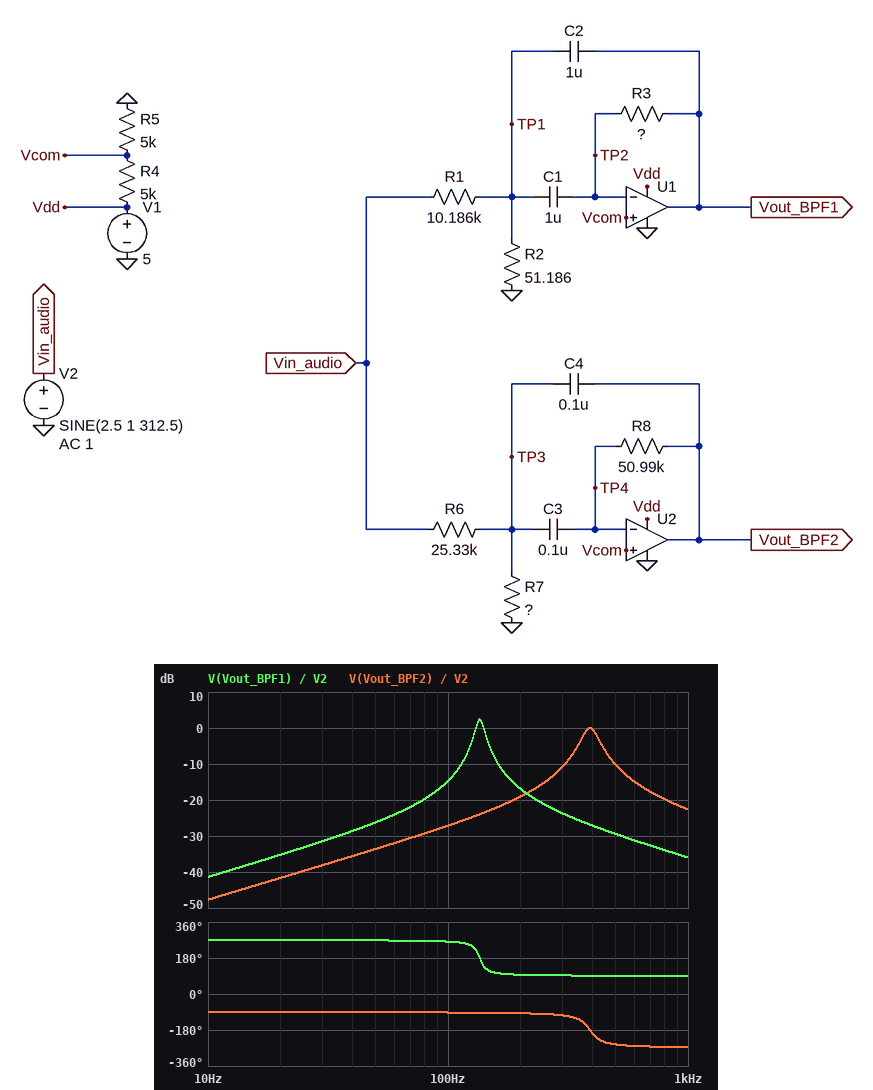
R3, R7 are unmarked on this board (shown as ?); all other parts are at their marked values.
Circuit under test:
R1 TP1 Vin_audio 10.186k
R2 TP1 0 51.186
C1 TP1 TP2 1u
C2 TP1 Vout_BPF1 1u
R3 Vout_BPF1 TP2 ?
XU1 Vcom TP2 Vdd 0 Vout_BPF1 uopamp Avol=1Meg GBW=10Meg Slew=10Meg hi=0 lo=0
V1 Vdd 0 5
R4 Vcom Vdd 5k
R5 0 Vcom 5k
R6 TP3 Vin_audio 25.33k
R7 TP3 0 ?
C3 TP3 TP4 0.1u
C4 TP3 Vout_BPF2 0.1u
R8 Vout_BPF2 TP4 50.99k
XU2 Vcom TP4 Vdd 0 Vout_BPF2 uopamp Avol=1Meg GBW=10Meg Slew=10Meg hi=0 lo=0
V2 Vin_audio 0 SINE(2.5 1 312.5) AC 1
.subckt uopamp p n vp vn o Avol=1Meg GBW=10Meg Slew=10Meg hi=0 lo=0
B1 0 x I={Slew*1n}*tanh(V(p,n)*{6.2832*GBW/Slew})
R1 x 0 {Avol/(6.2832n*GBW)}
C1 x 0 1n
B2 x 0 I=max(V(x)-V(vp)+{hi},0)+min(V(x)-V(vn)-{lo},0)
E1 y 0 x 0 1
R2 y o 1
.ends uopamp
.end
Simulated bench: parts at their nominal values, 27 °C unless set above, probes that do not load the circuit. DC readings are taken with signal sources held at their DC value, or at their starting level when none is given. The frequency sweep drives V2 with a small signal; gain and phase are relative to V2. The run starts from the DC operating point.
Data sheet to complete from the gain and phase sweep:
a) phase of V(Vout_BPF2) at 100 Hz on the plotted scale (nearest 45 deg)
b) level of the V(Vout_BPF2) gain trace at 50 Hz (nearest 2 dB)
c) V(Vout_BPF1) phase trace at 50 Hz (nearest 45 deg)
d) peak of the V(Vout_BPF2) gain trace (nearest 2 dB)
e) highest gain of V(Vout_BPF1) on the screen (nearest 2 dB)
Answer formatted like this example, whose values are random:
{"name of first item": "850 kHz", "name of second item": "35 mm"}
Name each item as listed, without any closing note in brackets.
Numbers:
{"phase of V(Vout_BPF2) at 100 Hz on the plotted scale": "-90 deg", "level of the V(Vout_BPF2) gain trace at 50 Hz": "-34 dB", "V(Vout_BPF1) phase trace at 50 Hz": "270 deg", "peak of the V(Vout_BPF2) gain trace": "0 dB", "highest gain of V(Vout_BPF1) on the screen": "2 dB"}
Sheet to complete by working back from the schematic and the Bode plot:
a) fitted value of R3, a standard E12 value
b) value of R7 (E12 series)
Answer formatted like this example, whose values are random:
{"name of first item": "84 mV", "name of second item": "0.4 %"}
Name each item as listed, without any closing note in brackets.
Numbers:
{"fitted value of R3, a standard E12 value": "27 kΩ", "value of R7": "330 Ω"}
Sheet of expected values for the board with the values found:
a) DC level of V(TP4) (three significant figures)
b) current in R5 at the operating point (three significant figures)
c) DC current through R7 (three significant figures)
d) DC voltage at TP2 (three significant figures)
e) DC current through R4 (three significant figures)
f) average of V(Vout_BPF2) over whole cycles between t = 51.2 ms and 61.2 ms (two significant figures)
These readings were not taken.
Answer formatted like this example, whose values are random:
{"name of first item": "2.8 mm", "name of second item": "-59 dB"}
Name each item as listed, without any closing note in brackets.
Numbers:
{"DC level of V(TP4)": "2.50 V", "current in R5 at the operating point": "500 µA", "DC current through R7": "97.4 µA", "DC voltage at TP2": "2.50 V", "DC current through R4": "500 µA", "average of V(Vout_BPF2) over whole cycles between t = 51.2 ms and 61.2 ms": "2.5 V"}
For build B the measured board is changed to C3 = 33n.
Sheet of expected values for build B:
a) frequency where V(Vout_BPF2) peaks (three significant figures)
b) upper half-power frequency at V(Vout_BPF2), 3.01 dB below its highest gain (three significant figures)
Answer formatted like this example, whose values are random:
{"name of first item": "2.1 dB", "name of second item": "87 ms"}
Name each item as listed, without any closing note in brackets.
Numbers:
{"frequency where V(Vout_BPF2) peaks": "680 Hz", "upper half-power frequency at V(Vout_BPF2), 3.01 dB below its highest gain": "745 Hz"}
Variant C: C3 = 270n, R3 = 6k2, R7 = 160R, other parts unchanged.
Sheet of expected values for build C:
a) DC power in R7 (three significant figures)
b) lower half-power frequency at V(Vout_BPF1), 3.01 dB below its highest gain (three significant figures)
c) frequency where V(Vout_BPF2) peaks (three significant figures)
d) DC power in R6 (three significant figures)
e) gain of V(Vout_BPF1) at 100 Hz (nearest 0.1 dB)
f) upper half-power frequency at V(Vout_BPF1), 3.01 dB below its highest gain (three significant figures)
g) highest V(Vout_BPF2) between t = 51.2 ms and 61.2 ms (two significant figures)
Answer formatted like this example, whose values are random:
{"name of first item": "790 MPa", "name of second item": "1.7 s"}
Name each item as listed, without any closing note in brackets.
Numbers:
{"DC power in R7": "1.54 µW", "lower half-power frequency at V(Vout_BPF1), 3.01 dB below its highest gain": "259 Hz", "frequency where V(Vout_BPF2) peaks": "340 Hz", "DC power in R6": "244 µW", "gain of V(Vout_BPF1) at 100 Hz": "-33.1 dB", "upper half-power frequency at V(Vout_BPF1), 3.01 dB below its highest gain": "310 Hz", "highest V(Vout_BPF2) between t = 51.2 ms and 61.2 ms": "3.4 V"}
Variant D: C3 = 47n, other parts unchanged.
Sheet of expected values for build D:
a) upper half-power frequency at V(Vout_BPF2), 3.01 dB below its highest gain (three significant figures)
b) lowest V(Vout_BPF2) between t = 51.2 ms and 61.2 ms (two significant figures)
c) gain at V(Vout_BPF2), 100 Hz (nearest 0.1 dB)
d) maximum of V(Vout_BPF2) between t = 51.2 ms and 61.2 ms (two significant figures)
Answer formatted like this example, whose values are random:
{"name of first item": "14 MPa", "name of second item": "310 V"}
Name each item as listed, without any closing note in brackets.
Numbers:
{"upper half-power frequency at V(Vout_BPF2), 3.01 dB below its highest gain": "620 Hz", "lowest V(Vout_BPF2) between t = 51.2 ms and 61.2 ms": "2.4 V", "gain at V(Vout_BPF2), 100 Hz": "-34.0 dB", "maximum of V(Vout_BPF2) between t = 51.2 ms and 61.2 ms": "2.6 V"}
